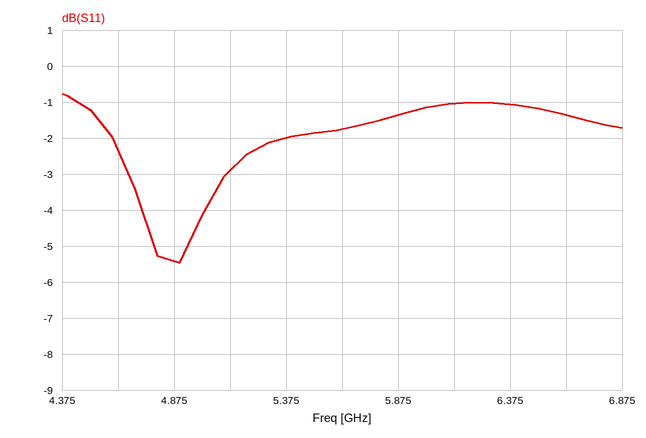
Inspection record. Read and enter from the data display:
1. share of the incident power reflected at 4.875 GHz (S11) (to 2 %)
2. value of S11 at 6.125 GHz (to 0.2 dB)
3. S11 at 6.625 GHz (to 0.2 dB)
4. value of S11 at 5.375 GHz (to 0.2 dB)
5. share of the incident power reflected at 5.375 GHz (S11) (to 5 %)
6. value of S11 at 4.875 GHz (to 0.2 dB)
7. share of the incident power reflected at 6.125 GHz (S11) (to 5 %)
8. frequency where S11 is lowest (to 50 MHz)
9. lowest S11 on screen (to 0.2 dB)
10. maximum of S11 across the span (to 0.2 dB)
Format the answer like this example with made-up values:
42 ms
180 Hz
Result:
28 %
-1.0 dB
-1.4 dB
-2.0 dB
65 %
-5.4 dB
80 %
4.90 GHz
-5.4 dB
-0.8 dB
